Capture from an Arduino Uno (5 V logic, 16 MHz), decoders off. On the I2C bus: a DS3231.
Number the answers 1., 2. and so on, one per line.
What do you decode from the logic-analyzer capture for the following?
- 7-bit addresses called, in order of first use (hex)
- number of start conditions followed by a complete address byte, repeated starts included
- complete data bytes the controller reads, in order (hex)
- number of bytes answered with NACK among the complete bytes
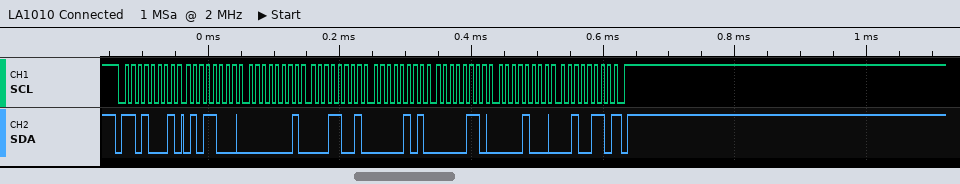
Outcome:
1. 0x68
2. 1
3. 58 01 19 05 06 08 26
4. 1
